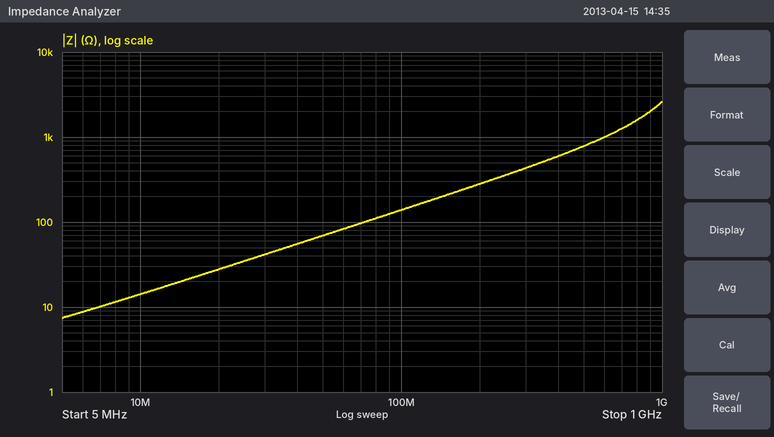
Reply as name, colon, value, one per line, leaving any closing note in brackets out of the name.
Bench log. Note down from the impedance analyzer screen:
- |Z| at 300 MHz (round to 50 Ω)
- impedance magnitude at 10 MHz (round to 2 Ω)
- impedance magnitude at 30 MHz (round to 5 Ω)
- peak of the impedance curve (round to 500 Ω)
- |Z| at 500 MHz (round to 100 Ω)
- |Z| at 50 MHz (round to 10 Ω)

|Z| at 300 MHz: 450 Ω
impedance magnitude at 10 MHz: 14 Ω
impedance magnitude at 30 MHz: 40 Ω
peak of the impedance curve: 2.5 kΩ
|Z| at 500 MHz: 800 Ω
|Z| at 50 MHz: 70 Ω
